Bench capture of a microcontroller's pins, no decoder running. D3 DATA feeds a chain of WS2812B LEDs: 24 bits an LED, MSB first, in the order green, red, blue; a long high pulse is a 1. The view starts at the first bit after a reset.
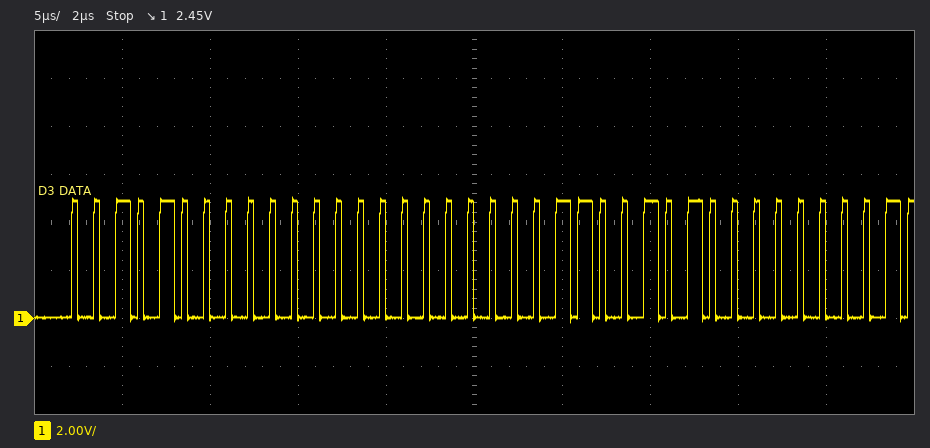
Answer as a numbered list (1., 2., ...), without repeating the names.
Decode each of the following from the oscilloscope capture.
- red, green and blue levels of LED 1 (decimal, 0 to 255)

1. 0, 40, 3
